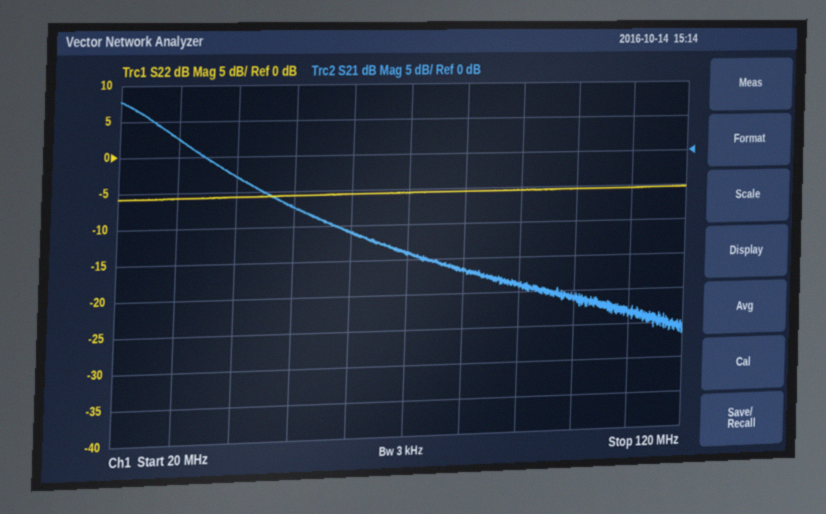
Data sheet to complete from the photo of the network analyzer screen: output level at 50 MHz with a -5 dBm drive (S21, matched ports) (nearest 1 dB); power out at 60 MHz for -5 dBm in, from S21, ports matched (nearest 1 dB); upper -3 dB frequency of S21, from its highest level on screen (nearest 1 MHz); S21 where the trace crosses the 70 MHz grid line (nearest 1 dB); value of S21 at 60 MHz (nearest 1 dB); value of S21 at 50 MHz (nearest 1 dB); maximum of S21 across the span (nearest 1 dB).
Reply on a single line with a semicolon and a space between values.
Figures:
-12 dBm; -16 dBm; 26 MHz; -14 dB; -11 dB; -7 dB; 8 dB
